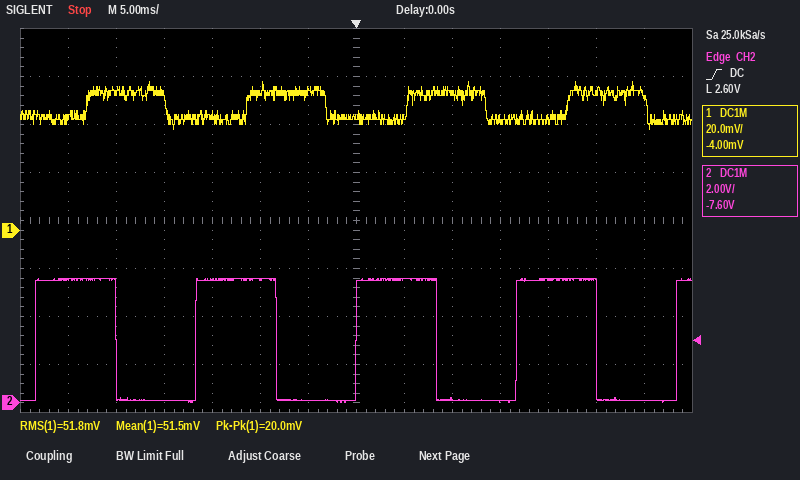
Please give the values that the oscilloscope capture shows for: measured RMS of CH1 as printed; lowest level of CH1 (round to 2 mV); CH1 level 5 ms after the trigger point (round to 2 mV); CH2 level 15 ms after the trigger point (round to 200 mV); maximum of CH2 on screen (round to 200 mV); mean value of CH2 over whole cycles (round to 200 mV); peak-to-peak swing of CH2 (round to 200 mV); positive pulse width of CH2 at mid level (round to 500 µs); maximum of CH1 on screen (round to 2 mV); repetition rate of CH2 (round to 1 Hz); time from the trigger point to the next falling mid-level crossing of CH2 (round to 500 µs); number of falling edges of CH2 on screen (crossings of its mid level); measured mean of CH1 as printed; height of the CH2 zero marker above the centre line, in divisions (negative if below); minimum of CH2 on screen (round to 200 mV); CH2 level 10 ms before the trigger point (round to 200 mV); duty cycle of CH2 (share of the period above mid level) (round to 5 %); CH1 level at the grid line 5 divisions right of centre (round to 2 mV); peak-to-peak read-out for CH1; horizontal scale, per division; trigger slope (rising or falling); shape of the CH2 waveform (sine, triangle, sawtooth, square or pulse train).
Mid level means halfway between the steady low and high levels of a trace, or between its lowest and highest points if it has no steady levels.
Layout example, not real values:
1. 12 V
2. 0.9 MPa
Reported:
1. 51.8 mV
2. 42 mV
3. 46 mV
4. 0.0 V
5. 5.2 V
6. 2.6 V
7. 5.2 V
8. 8.5 ms
9. 62 mV
10. 60 Hz
11. 8.5 ms
12. 4
13. 51.5 mV
14. -3.8 div
15. 0.0 V
16. 5.2 V
17. 50 %
18. 58 mV
19. 20.0 mV
20. 5 ms
21. rising
22. square
